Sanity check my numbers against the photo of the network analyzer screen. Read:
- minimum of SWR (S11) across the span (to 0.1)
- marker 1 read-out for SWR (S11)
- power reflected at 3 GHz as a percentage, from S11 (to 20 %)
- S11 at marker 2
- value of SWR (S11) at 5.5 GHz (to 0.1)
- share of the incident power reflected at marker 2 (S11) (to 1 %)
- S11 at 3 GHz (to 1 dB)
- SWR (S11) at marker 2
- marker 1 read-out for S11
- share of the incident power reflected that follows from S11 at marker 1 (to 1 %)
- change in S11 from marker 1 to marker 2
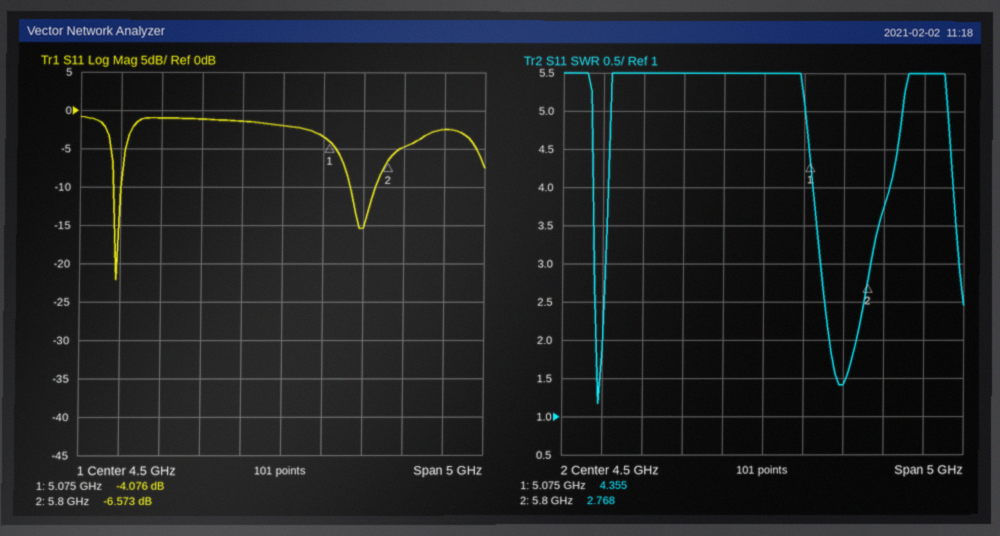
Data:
1.2
4.355
80 %
-6.573 dB
1.4
22 %
-1 dB
2.768
-4.076 dB
39 %
-2.497 dB
